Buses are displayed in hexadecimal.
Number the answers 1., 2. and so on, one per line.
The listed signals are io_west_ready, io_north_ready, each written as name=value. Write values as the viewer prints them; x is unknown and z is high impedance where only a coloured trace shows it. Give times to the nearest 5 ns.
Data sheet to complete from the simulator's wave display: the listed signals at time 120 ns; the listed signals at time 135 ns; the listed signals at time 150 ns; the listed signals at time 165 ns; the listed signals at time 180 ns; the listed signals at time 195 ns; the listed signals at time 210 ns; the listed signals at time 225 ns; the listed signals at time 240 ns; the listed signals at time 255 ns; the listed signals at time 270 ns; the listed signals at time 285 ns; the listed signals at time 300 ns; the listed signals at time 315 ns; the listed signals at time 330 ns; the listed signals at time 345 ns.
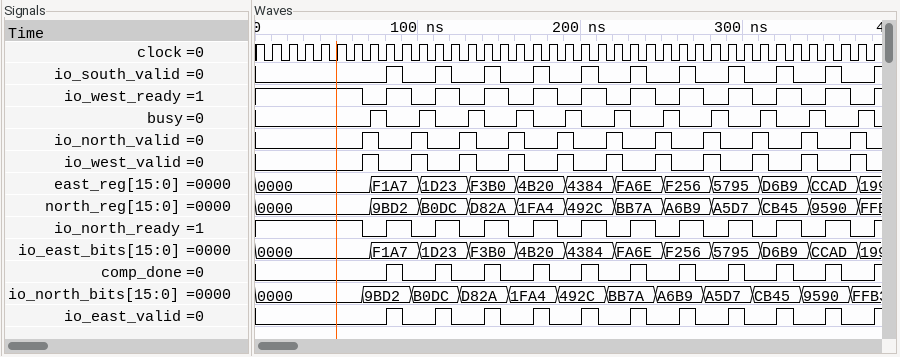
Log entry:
1. io_west_ready=1, io_north_ready=1
2. io_west_ready=0, io_north_ready=0
3. io_west_ready=1, io_north_ready=1
4. io_west_ready=0, io_north_ready=0
5. io_west_ready=1, io_north_ready=1
6. io_west_ready=0, io_north_ready=0
7. io_west_ready=1, io_north_ready=1
8. io_west_ready=0, io_north_ready=0
9. io_west_ready=1, io_north_ready=1
10. io_west_ready=0, io_north_ready=0
11. io_west_ready=1, io_north_ready=1
12. io_west_ready=0, io_north_ready=0
13. io_west_ready=1, io_north_ready=1
14. io_west_ready=0, io_north_ready=0
15. io_west_ready=1, io_north_ready=1
16. io_west_ready=0, io_north_ready=0
